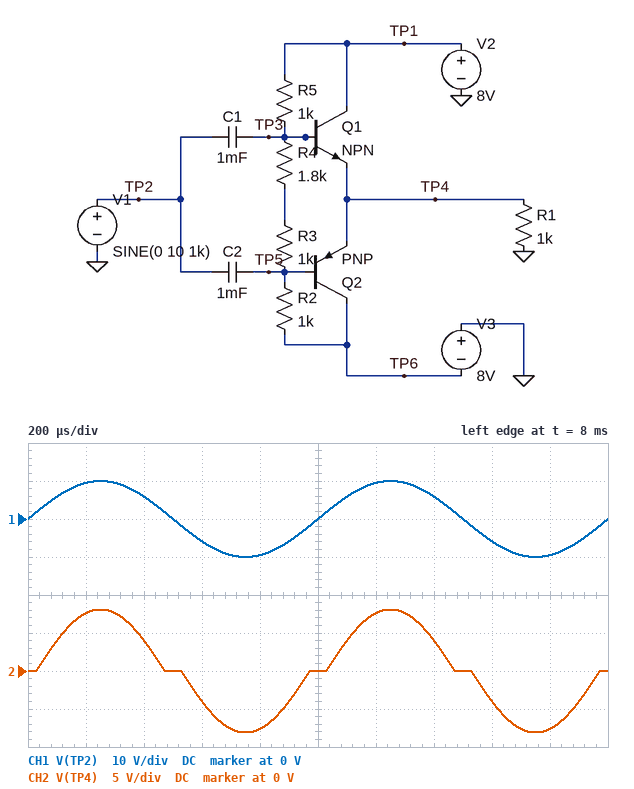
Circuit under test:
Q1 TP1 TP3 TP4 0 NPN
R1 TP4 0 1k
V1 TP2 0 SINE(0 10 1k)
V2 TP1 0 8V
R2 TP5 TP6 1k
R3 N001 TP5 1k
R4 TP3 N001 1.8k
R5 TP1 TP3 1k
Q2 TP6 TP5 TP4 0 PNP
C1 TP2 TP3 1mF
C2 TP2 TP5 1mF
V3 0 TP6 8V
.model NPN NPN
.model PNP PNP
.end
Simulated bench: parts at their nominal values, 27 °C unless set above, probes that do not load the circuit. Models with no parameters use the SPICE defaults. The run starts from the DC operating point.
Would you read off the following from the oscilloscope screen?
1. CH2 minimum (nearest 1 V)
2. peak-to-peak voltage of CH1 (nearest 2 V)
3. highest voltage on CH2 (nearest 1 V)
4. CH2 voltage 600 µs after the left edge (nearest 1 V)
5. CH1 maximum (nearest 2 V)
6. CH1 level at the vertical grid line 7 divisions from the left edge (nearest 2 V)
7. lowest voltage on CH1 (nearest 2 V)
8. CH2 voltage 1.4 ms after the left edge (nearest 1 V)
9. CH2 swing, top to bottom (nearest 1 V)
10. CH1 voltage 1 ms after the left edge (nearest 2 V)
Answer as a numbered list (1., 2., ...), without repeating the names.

1. -8 V
2. 20 V
3. 8 V
4. -4 V
5. 10 V
6. 6 V
7. -10 V
8. 4 V
9. 16 V
10. 0 V
